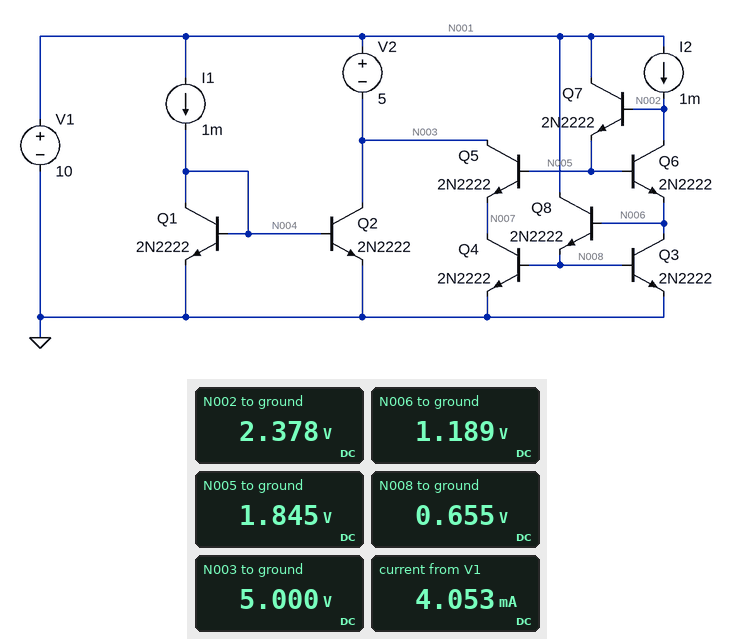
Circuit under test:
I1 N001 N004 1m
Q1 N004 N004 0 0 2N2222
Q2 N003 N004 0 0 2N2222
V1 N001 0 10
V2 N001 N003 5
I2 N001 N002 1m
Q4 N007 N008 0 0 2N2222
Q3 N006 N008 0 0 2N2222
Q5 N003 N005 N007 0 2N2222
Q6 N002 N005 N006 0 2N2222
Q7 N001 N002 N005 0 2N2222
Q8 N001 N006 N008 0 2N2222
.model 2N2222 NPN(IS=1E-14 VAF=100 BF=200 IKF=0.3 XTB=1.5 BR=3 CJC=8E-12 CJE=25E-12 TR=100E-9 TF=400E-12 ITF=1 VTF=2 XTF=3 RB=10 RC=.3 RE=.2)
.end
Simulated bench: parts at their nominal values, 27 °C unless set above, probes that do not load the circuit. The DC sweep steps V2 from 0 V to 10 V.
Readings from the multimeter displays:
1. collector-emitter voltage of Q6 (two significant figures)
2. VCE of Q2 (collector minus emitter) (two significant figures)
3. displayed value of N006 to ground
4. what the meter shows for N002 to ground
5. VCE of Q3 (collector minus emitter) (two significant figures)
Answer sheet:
1.2 V
5.0 V
1.189 V
2.378 V
1.2 V
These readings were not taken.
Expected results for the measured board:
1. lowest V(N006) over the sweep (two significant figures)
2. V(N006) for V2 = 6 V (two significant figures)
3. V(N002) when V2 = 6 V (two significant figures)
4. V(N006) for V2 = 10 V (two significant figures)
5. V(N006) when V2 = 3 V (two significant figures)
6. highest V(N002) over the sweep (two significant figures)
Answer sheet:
1.2 V
1.2 V
2.4 V
1.2 V
1.2 V
2.6 V
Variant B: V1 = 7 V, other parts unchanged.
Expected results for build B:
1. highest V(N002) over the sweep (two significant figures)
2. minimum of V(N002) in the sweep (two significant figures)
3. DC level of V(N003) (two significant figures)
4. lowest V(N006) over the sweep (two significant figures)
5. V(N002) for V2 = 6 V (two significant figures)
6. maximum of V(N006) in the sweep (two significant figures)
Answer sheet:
2.7 V
100 mV
2.0 V
-1.3 V
2.6 V
1.3 V
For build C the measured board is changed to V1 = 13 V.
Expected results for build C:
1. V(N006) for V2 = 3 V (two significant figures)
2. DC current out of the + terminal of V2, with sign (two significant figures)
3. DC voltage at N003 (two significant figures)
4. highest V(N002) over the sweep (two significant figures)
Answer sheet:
1.2 V
-2.1 mA
8.0 V
2.4 V
